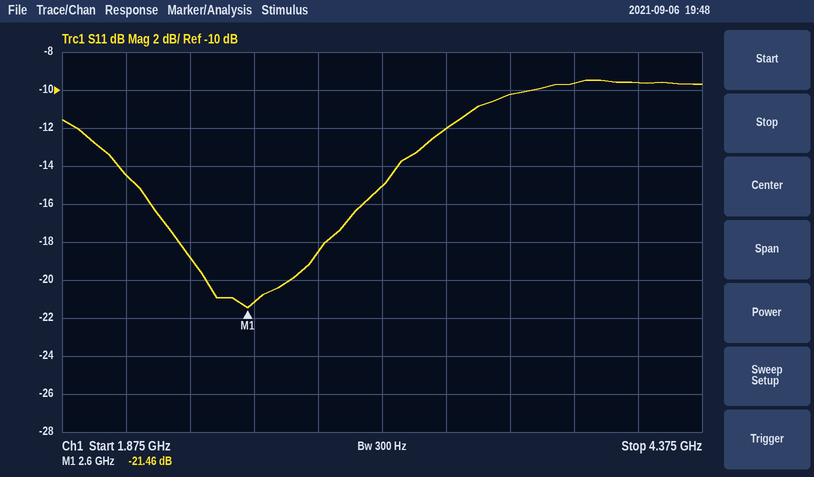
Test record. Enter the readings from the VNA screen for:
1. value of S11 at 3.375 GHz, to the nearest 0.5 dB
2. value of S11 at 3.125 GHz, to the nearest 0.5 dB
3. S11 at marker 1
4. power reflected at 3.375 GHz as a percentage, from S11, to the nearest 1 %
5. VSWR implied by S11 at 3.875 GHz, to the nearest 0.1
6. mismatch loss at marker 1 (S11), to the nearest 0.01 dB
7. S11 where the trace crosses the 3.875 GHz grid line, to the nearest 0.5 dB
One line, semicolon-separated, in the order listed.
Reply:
-12.0 dB; -15.0 dB; -21.46 dB; 6 %; 2.0; 0.03 dB; -9.5 dB
